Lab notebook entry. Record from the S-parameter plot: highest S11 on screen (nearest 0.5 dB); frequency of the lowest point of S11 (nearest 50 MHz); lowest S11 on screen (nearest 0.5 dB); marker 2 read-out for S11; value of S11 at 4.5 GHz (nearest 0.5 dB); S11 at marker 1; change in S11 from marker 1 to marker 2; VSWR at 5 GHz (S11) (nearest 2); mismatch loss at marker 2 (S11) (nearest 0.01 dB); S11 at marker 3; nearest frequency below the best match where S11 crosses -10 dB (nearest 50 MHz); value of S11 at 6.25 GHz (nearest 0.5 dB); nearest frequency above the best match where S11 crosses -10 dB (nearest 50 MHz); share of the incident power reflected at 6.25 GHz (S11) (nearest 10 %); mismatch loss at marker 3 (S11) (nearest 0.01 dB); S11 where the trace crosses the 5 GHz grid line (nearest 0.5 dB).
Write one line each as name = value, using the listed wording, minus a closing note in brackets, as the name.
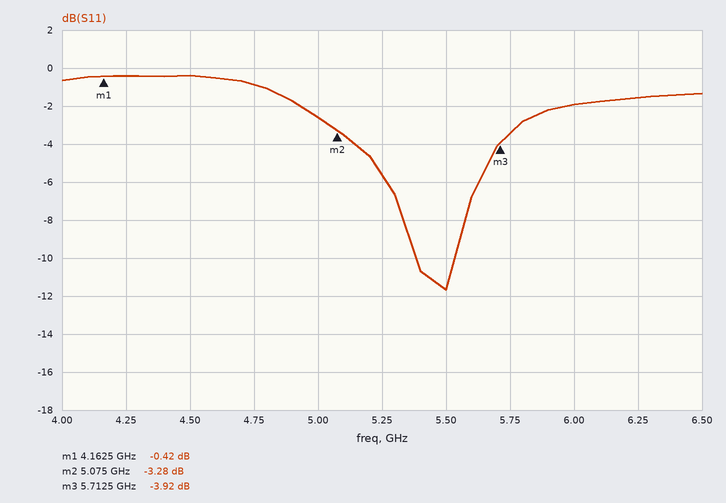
highest S11 on screen = -0.5 dB
frequency of the lowest point of S11 = 5.50 GHz
lowest S11 on screen = -11.5 dB
marker 2 read-out for S11 = -3.28 dB
value of S11 at 4.5 GHz = -0.5 dB
S11 at marker 1 = -0.42 dB
change in S11 from marker 1 to marker 2 = -2.86 dB
VSWR at 5 GHz (S11) = 6
mismatch loss at marker 2 (S11) = 2.76 dB
S11 at marker 3 = -3.92 dB
nearest frequency below the best match where S11 crosses -10 dB = 5.40 GHz
value of S11 at 6.25 GHz = -1.5 dB
nearest frequency above the best match where S11 crosses -10 dB = 5.55 GHz
share of the incident power reflected at 6.25 GHz (S11) = 70 %
mismatch loss at marker 3 (S11) = 2.26 dB
S11 where the trace crosses the 5 GHz grid line = -2.5 dB
